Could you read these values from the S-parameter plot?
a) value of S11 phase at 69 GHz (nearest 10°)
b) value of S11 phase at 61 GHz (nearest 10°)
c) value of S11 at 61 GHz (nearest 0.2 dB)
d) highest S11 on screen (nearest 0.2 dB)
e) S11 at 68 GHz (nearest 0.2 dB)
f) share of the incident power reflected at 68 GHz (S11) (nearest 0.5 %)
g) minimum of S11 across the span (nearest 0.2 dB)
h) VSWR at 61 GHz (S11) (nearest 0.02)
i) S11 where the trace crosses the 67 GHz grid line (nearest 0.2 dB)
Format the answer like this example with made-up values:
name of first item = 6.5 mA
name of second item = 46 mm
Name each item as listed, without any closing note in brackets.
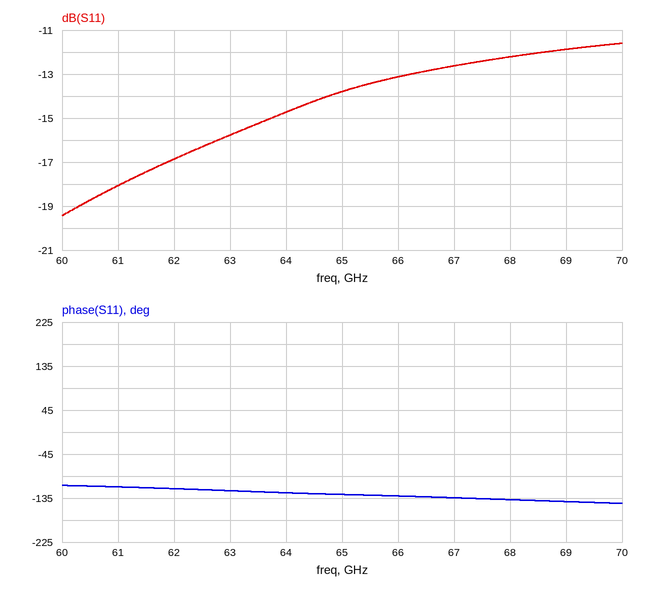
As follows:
value of S11 phase at 69 GHz = -140°
value of S11 phase at 61 GHz = -110°
value of S11 at 61 GHz = -18.0 dB
highest S11 on screen = -11.6 dB
S11 at 68 GHz = -12.2 dB
share of the incident power reflected at 68 GHz (S11) = 6.0 %
minimum of S11 across the span = -19.4 dB
VSWR at 61 GHz (S11) = 1.28
S11 where the trace crosses the 67 GHz grid line = -12.6 dB
